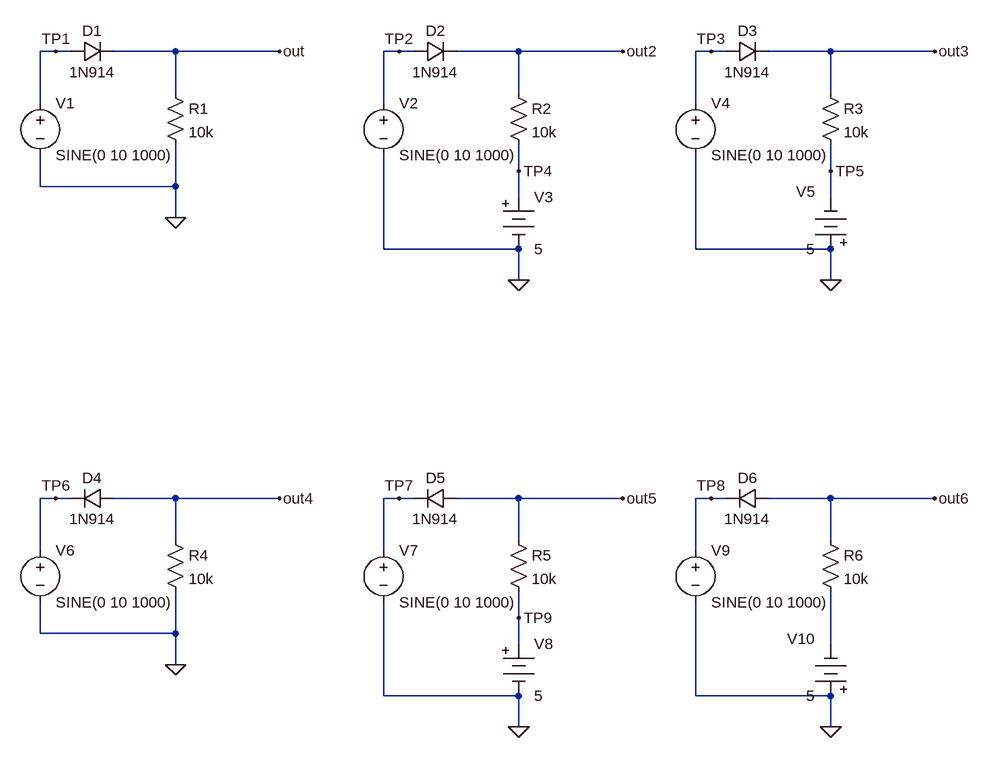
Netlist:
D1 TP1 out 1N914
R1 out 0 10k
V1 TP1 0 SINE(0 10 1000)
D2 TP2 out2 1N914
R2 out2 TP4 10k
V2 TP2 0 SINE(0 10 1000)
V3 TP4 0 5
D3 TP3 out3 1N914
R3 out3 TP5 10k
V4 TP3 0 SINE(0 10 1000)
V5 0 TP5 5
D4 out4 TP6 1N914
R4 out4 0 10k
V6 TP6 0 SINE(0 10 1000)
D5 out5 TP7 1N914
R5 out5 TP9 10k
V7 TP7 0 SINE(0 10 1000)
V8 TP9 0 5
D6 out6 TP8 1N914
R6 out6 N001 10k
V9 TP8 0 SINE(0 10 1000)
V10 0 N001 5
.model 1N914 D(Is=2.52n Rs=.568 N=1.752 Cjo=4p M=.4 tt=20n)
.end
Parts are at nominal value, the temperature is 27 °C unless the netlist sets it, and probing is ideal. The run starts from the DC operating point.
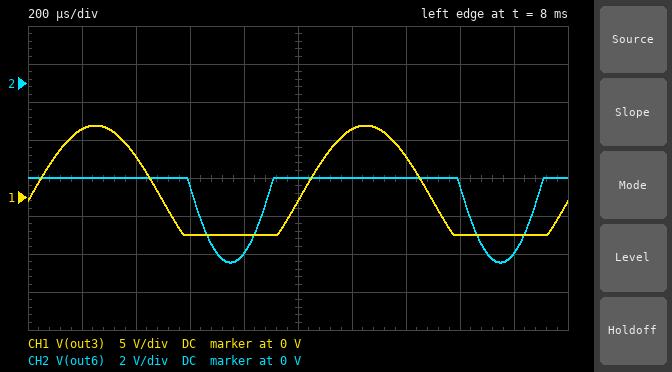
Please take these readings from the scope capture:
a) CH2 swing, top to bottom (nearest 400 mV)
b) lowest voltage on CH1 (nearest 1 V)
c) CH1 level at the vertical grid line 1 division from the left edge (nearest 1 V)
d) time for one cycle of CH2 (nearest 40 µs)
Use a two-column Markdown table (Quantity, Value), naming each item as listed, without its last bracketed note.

| Quantity | Value |
|---|---|
| CH2 swing, top to bottom | 4.4 V |
| lowest voltage on CH1 | -5 V |
| CH1 level at the vertical grid line 1 division from the left edge | 9 V |
| time for one cycle of CH2 | 1.00 ms |
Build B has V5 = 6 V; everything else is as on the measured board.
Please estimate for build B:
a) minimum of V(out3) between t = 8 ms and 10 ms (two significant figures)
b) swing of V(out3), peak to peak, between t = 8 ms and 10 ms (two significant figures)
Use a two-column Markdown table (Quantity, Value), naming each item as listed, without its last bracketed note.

| Quantity | Value |
|---|---|
| minimum of V(out3) between t = 8 ms and 10 ms | -6.0 V |
| swing of V(out3), peak to peak, between t = 8 ms and 10 ms | 15 V |
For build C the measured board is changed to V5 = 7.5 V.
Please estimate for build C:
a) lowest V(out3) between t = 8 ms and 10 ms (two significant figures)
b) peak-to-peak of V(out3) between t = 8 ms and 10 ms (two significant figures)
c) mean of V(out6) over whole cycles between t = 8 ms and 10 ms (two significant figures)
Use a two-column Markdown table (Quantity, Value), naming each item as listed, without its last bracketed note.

| Quantity | Value |
|---|---|
| lowest V(out3) between t = 8 ms and 10 ms | -7.5 V |
| peak-to-peak of V(out3) between t = 8 ms and 10 ms | 17 V |
| mean of V(out6) over whole cycles between t = 8 ms and 10 ms | -5.9 V |
